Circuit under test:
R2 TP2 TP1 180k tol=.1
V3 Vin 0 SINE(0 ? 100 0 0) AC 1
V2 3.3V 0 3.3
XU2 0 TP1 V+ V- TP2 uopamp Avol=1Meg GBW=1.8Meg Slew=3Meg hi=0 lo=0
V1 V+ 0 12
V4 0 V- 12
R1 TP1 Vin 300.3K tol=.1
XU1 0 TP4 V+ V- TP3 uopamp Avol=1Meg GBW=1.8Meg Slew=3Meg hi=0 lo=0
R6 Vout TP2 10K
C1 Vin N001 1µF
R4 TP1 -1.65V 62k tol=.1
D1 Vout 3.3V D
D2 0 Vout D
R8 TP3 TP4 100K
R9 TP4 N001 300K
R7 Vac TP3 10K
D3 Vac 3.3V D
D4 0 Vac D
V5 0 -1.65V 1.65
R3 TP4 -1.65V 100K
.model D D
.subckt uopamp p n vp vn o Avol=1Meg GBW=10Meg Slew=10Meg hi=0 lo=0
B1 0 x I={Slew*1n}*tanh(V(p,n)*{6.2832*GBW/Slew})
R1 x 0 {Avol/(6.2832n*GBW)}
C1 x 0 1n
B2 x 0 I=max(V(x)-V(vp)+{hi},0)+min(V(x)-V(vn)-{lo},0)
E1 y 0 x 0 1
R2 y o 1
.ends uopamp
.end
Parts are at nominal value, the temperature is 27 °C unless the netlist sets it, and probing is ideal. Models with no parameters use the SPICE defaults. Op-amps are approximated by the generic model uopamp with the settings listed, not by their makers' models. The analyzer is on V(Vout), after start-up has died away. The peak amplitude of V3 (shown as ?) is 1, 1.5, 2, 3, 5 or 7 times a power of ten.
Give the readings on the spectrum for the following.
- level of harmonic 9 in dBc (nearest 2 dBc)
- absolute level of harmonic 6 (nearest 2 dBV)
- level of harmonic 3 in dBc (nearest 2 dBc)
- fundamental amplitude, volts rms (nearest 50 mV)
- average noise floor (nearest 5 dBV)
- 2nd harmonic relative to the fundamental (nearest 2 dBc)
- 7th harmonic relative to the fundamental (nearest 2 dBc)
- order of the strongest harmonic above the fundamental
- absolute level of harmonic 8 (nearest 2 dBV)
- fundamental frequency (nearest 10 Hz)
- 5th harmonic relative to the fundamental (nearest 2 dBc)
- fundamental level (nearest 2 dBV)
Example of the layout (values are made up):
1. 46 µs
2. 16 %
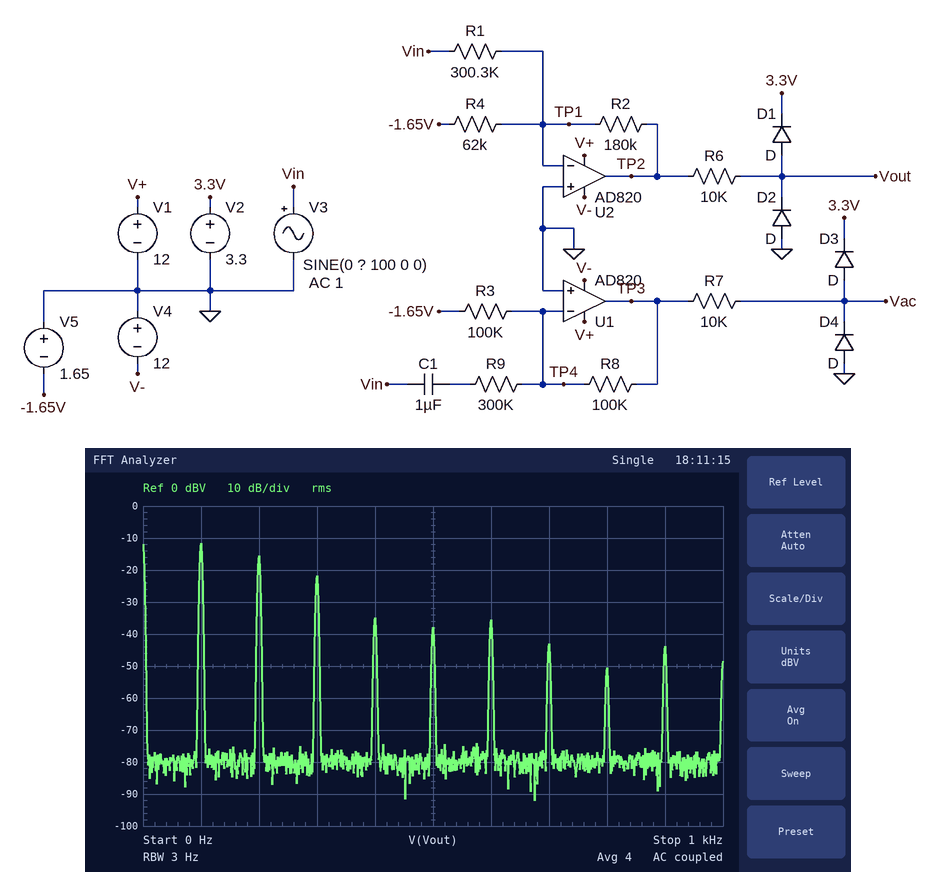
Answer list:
1. -32 dBc
2. -36 dBV
3. -10 dBc
4. 250 mV
5. -80 dBV
6. -4 dBc
7. -32 dBc
8. 2
9. -50 dBV
10. 100 Hz
11. -26 dBc
12. -12 dBV
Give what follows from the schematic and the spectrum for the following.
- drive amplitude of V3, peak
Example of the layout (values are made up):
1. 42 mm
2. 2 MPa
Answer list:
1. 3 V
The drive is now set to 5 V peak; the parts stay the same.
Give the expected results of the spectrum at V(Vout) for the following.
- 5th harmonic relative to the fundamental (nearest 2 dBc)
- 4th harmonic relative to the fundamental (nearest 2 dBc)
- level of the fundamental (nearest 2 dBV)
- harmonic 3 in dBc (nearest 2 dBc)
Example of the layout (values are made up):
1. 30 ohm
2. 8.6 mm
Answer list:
1. -22 dBc
2. -26 dBc
3. -4 dBV
4. -16 dBc
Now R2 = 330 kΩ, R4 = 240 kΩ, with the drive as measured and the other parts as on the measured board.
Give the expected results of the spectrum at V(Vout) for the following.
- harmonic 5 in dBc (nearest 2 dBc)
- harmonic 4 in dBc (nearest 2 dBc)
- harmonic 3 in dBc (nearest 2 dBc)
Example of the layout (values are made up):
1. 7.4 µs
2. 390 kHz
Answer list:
1. -54 dBc
2. -40 dBc
3. -18 dBc
